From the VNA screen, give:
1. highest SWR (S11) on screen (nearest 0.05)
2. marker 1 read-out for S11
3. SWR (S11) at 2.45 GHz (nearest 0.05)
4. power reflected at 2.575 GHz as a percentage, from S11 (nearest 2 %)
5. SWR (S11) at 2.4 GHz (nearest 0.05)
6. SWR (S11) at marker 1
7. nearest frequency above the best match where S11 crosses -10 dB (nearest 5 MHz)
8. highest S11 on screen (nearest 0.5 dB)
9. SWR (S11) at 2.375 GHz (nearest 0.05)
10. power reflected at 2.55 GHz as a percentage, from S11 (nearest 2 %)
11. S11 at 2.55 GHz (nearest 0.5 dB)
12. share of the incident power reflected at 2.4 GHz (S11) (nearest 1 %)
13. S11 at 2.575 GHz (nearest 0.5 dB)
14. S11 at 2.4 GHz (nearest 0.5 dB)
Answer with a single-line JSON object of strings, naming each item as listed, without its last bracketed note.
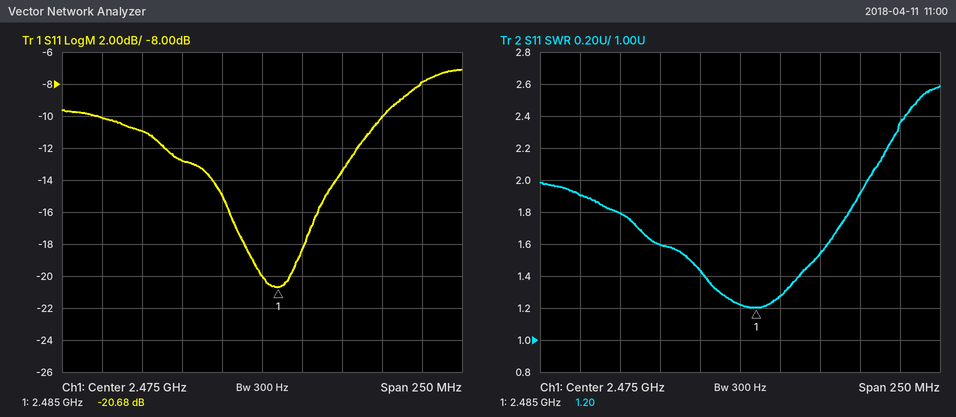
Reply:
{"highest SWR (S11) on screen": "2.60", "marker 1 read-out for S11": "-20.68 dB", "SWR (S11) at 2.45 GHz": "1.45", "power reflected at 2.575 GHz as a percentage, from S11": "16 %", "SWR (S11) at 2.4 GHz": "1.80", "SWR (S11) at marker 1": "1.20", "nearest frequency above the best match where S11 crosses -10 dB": "2.550 GHz", "highest S11 on screen": "-7.0 dB", "SWR (S11) at 2.375 GHz": "1.90", "power reflected at 2.55 GHz as a percentage, from S11": "10 %", "S11 at 2.55 GHz": "-10.0 dB", "share of the incident power reflected at 2.4 GHz (S11)": "8 %", "S11 at 2.575 GHz": "-8.0 dB", "S11 at 2.4 GHz": "-11.0 dB"}
